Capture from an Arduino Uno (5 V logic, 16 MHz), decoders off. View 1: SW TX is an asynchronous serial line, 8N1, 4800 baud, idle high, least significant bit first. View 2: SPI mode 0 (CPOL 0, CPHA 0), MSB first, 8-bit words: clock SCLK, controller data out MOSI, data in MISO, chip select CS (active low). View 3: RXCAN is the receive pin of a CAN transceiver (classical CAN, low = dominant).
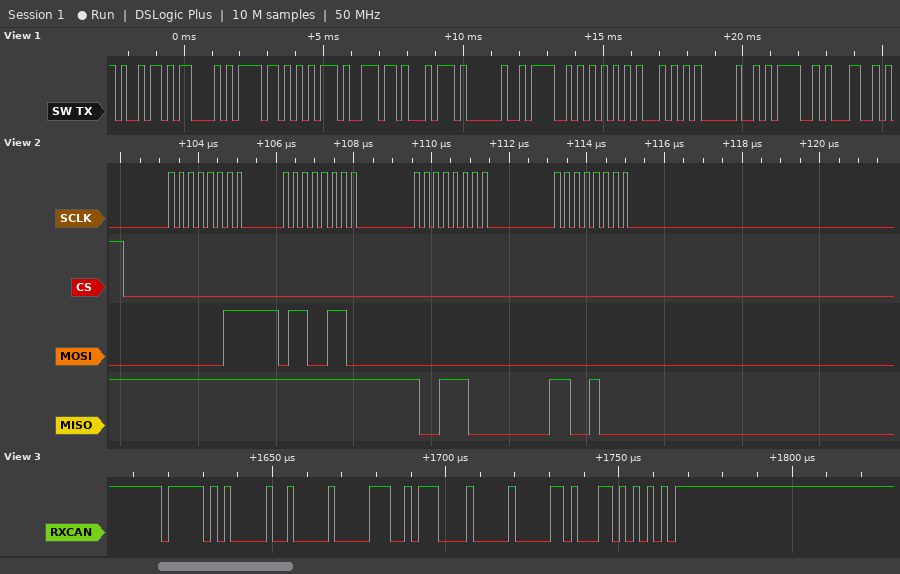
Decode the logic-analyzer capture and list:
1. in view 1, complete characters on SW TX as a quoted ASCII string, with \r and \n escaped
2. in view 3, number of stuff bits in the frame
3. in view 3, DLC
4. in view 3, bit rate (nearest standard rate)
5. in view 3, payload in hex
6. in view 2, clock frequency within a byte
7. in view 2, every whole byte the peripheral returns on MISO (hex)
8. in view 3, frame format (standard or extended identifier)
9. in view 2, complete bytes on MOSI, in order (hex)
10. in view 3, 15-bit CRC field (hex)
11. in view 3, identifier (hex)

"iCount OUT =1"
6
4
500 kbit/s
00 CB 84 00
4 MHz
FF FF 9C C8
standard
03 66 00 00
0x51AA
0x7E8
